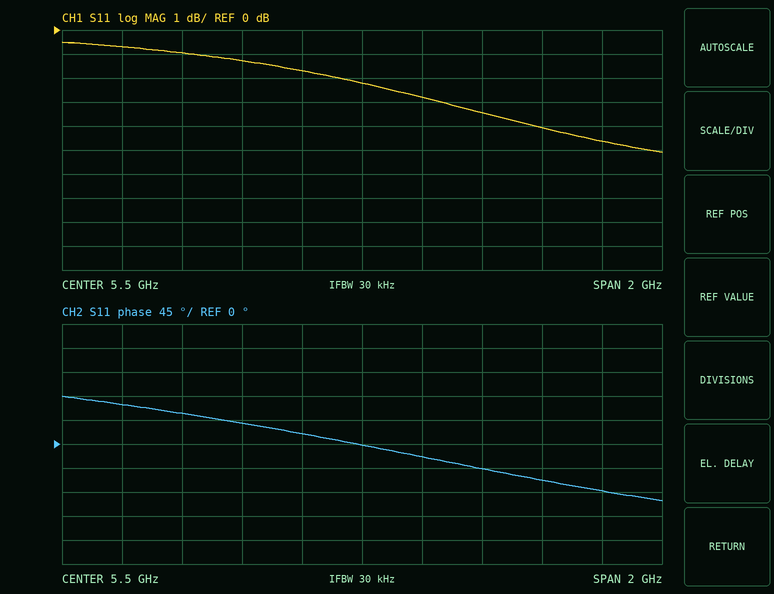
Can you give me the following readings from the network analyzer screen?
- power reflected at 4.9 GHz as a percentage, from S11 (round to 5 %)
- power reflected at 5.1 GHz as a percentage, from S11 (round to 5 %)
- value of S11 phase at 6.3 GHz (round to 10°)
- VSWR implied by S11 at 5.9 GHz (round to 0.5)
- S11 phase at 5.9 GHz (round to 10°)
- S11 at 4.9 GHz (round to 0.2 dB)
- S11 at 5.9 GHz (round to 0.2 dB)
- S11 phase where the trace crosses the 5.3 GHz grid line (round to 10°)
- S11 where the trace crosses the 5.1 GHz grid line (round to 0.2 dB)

80 %
75 %
-90°
5.0
-50°
-1.0 dB
-3.4 dB
20°
-1.2 dB
